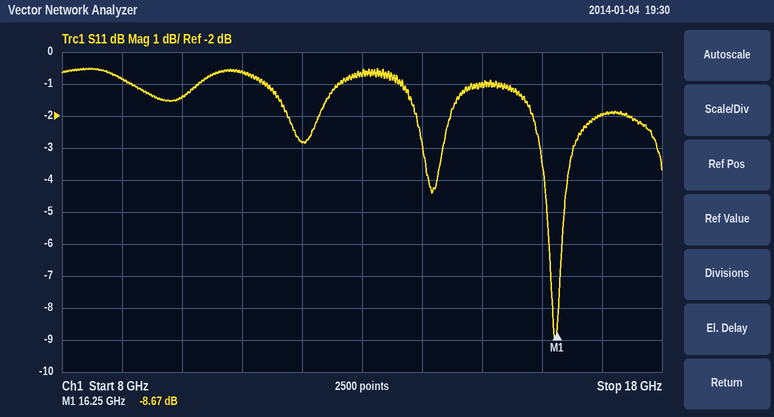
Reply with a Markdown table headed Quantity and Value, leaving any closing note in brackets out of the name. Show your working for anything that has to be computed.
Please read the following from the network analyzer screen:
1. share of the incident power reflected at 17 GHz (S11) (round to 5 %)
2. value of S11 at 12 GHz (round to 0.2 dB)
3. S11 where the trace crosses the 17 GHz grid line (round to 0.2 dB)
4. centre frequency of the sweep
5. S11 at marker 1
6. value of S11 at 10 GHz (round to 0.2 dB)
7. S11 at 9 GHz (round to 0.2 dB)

| Quantity | Value |
|---|---|
| share of the incident power reflected at 17 GHz (S11) | 10^(-2/10) ≈ 63.1 %, so 65 % to the nearest 5 % |
| value of S11 at 12 GHz | -2.8 dB |
| S11 where the trace crosses the 17 GHz grid line | -2.0 dB |
| centre frequency of the sweep | 13 GHz |
| S11 at marker 1 | -8.67 dB |
| value of S11 at 10 GHz | -1.4 dB |
| S11 at 9 GHz | -0.8 dB |
